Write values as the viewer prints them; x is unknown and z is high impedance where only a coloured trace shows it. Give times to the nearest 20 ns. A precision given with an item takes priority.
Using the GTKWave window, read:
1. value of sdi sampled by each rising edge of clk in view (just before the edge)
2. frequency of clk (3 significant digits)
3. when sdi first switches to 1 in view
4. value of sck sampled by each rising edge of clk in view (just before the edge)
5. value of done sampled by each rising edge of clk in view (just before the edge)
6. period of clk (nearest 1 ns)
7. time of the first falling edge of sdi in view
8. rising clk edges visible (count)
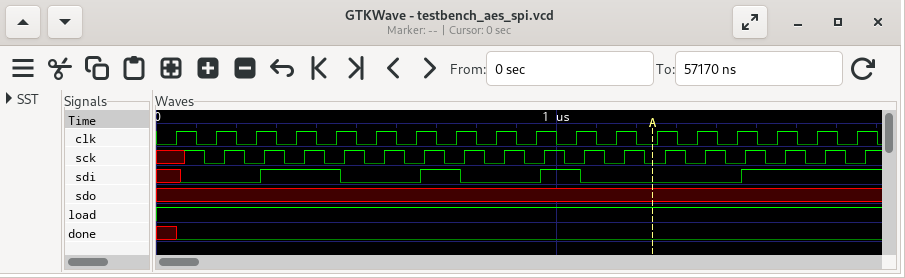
x 0 0 1 1 0 0 1 0 0 1 0 0 0 0 1 1 1
10.0 MHz
260 ns
x 0 0 0 0 0 0 0 0 0 0 0 0 0 0 0 0 0
x 0 0 0 0 0 0 0 0 0 0 0 0 0 0 0 0 0
100 ns
460 ns
18
